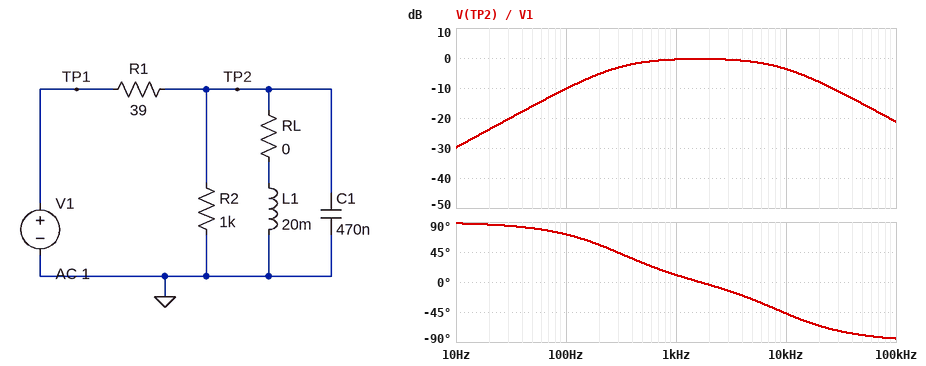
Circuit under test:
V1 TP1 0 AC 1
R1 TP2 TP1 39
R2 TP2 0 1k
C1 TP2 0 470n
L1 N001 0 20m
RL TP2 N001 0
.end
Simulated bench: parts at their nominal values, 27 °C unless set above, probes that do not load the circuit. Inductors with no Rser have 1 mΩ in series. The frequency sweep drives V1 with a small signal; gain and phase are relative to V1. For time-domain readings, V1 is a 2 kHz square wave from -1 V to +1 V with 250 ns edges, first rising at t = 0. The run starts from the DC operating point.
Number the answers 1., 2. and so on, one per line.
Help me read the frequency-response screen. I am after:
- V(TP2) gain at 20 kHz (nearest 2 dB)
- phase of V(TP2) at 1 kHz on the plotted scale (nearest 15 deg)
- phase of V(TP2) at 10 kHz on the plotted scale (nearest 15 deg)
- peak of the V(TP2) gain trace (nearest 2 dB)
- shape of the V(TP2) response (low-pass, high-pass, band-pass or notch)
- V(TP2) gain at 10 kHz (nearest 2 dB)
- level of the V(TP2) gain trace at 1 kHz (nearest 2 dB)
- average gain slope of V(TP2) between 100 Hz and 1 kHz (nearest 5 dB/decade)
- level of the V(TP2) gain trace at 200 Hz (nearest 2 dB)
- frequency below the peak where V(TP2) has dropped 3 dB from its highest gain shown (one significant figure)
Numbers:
1. -8 dB
2. 15 deg
3. -45 deg
4. 0 dB
5. band-pass
6. -4 dB
7. 0 dB
8. 10 dB/decade
9. -6 dB
10. 300 Hz
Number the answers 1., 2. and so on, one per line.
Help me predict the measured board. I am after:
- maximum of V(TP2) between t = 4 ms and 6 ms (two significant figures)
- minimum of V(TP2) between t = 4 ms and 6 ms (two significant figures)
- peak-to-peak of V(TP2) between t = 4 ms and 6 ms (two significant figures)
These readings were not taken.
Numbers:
1. 1.1 V
2. -1.1 V
3. 2.1 V
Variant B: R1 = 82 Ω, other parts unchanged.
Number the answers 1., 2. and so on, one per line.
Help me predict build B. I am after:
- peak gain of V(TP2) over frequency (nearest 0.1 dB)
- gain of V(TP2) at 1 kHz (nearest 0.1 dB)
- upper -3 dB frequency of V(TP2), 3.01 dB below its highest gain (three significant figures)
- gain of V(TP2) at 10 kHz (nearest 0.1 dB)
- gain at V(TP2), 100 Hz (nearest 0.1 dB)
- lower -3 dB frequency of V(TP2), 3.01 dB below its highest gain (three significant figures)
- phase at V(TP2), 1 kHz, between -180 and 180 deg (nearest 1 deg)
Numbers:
1. -0.6 dB
2. -1.2 dB
3. 4.97 kHz
4. -8.3 dB
5. -16.4 dB
6. 543 Hz
7. 21 deg
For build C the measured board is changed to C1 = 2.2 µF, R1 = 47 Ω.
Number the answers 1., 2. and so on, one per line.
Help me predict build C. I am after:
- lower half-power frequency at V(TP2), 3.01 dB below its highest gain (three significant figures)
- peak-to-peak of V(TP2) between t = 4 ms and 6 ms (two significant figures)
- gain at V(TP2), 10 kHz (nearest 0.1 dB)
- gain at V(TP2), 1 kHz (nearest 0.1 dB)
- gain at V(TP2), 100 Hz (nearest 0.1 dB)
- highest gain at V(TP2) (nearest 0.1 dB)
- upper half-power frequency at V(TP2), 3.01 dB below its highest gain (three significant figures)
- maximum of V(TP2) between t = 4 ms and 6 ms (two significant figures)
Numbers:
1. 302 Hz
2. 1.7 V
3. -16.3 dB
4. -0.7 dB
5. -11.6 dB
6. -0.4 dB
7. 1.91 kHz
8. 830 mV
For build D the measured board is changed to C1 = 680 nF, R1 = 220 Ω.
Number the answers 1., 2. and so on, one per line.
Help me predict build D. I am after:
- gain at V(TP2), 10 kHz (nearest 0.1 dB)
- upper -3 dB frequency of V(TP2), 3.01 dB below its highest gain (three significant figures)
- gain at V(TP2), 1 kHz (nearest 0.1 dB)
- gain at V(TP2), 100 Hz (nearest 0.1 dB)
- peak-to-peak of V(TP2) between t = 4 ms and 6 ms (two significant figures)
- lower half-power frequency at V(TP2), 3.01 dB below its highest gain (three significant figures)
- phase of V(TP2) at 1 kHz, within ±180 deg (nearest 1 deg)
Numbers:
1. -19.4 dB
2. 2.15 kHz
3. -3.3 dB
4. -24.8 dB
5. 1.5 V
6. 866 Hz
7. 34 deg
